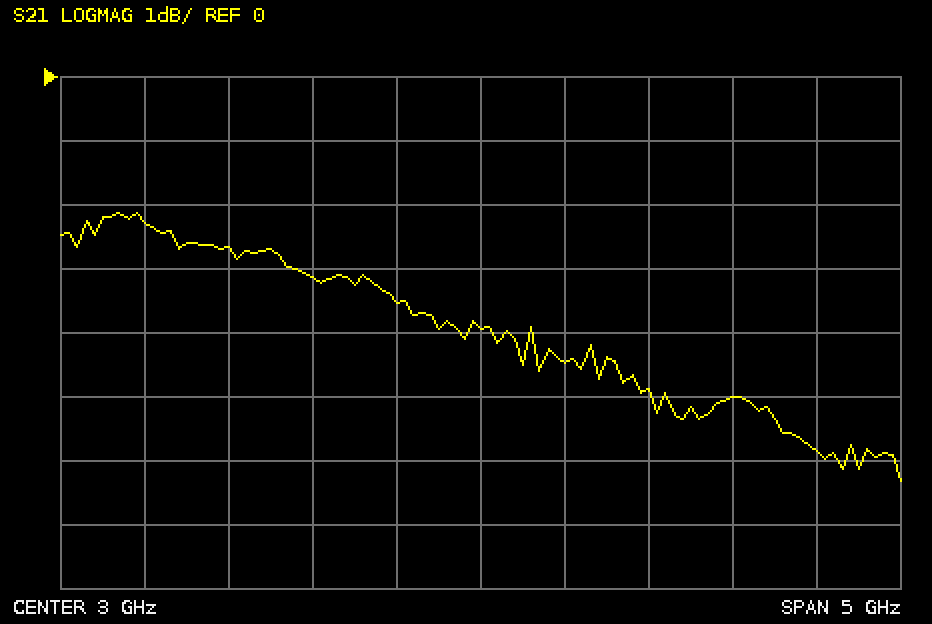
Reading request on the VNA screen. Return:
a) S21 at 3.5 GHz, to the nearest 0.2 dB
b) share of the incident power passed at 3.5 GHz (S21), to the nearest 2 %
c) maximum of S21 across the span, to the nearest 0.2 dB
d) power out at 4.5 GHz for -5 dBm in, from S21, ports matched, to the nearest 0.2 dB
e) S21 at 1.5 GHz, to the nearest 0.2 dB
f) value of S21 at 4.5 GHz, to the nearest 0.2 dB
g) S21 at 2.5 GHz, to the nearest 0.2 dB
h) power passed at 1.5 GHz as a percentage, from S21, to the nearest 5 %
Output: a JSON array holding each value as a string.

["-4.4 dB", "36 %", "-2.2 dB", "-10.0 dBm", "-2.6 dB", "-5.0 dB", "-3.6 dB", "55 %"]
